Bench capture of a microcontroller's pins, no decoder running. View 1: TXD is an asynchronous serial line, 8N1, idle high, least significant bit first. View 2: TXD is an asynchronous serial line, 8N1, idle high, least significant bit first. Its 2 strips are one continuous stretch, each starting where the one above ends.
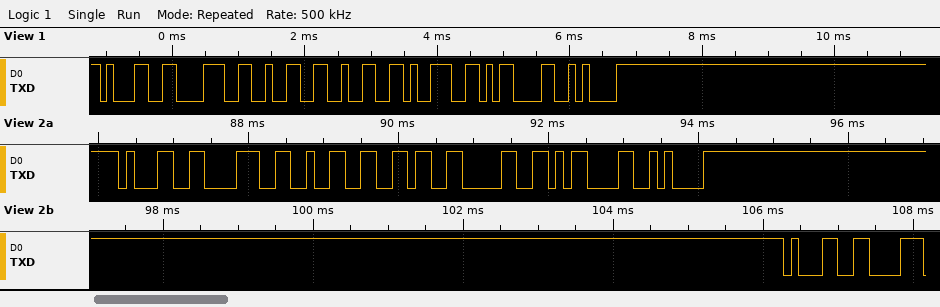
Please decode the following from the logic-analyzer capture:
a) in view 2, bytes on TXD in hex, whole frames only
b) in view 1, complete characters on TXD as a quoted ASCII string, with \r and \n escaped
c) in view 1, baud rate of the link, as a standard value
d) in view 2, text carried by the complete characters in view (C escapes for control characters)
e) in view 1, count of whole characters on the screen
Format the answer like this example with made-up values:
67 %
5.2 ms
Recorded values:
31 38 32 36 30 0D 0A 31
"18229\r\n"
9600 baud
"18260\r\n1"
7
